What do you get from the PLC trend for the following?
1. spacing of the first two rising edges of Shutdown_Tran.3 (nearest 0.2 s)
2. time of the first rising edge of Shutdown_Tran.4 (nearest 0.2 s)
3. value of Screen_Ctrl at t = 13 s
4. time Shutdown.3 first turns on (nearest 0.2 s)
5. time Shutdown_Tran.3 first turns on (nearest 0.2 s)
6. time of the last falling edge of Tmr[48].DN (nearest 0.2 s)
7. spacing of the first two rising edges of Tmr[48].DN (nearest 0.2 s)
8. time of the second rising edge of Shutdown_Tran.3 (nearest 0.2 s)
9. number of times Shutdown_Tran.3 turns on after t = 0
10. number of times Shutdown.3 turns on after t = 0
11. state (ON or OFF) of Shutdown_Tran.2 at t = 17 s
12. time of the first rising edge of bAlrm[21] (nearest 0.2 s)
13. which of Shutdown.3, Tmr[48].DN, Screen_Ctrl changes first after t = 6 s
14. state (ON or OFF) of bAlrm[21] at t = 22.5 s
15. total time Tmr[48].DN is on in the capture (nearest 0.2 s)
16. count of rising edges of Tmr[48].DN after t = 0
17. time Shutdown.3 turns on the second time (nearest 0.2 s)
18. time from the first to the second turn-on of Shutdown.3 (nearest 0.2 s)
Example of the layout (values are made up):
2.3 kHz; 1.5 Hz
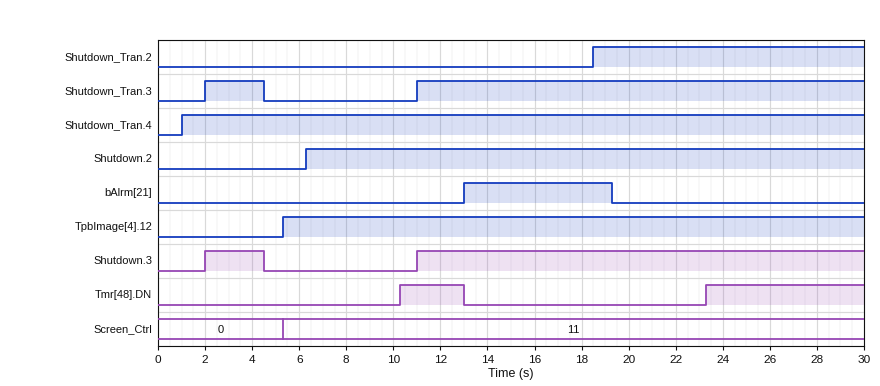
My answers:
9.0 s; 1.0 s; 11; 2.0 s; 2.0 s; 13.0 s; 13.0 s; 11.0 s; 2; 2; OFF; 13.0 s; Tmr[48].DN; OFF; 9.4 s; 2; 11.0 s; 9.0 s
